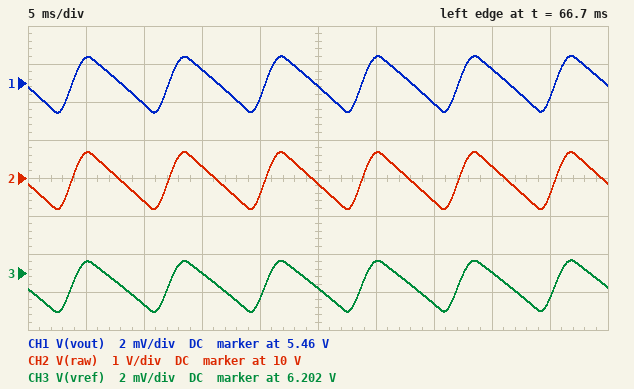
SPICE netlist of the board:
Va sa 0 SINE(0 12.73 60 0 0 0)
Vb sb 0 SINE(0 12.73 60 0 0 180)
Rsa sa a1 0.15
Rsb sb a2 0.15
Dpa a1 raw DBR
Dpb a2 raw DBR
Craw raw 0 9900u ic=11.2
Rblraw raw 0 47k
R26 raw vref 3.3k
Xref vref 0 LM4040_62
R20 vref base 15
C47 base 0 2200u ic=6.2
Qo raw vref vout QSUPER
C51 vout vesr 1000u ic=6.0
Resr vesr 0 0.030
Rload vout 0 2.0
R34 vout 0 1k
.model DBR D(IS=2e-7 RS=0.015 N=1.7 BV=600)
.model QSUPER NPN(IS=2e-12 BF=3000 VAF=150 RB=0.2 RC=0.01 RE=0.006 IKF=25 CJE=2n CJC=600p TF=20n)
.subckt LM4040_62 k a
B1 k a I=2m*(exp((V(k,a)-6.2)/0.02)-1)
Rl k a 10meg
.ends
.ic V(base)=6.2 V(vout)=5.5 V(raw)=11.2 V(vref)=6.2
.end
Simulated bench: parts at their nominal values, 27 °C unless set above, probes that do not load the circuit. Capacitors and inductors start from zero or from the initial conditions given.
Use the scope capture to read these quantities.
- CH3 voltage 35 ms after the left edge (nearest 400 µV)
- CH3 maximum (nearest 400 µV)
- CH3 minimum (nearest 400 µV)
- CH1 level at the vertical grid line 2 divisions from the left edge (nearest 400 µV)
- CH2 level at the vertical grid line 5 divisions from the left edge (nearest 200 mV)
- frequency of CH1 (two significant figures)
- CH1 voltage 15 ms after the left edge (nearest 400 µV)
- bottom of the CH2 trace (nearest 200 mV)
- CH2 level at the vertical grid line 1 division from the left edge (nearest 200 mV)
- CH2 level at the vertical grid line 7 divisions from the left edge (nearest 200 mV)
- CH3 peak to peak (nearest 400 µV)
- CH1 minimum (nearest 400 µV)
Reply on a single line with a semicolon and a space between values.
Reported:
6.2004 V; 6.2028 V; 6.2000 V; 5.4588 V; 9.8 V; 120 Hz; 5.4608 V; 9.2 V; 10.6 V; 9.4 V; 2.8 mV; 5.4584 V
